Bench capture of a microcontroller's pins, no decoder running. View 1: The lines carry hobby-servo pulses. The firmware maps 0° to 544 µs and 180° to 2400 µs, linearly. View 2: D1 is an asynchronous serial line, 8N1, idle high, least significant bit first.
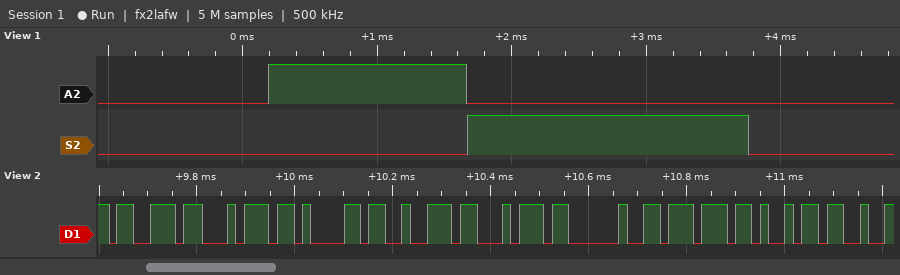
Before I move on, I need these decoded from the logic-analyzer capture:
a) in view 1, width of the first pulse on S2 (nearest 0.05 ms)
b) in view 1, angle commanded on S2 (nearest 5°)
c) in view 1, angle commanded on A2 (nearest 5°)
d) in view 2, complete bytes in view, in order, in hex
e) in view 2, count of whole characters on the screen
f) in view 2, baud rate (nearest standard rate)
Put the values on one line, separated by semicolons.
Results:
2.10 ms; 150°; 90°; 73 74 61 72 74 20 77 69; 8; 57600 baud
